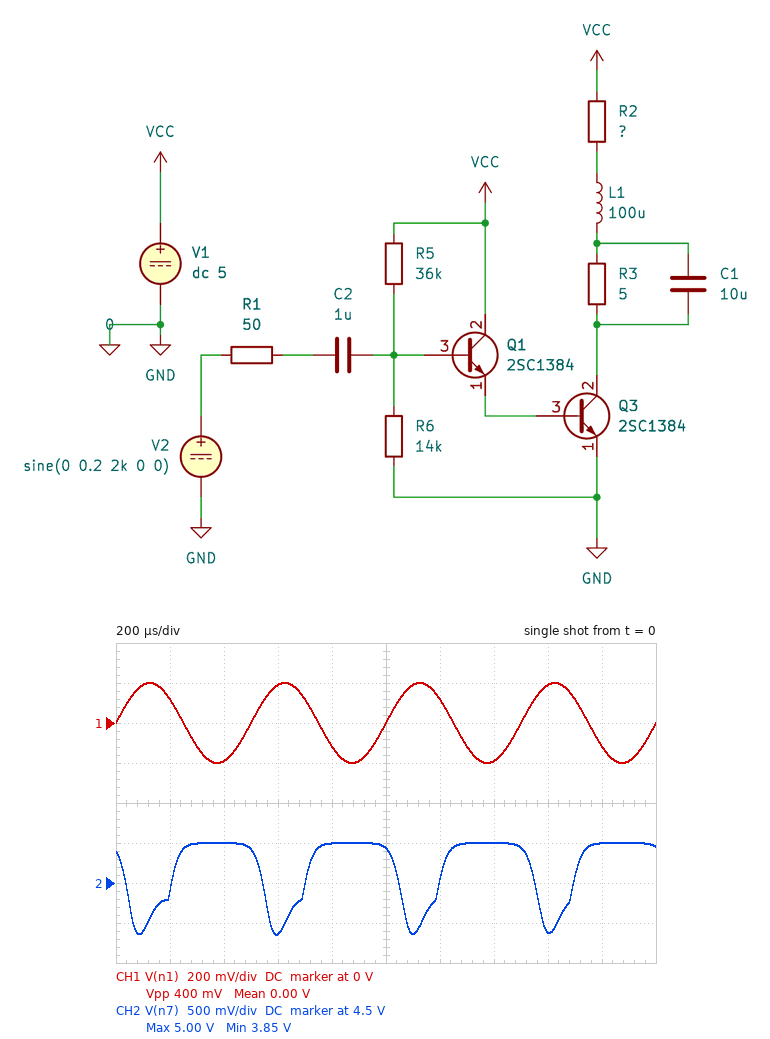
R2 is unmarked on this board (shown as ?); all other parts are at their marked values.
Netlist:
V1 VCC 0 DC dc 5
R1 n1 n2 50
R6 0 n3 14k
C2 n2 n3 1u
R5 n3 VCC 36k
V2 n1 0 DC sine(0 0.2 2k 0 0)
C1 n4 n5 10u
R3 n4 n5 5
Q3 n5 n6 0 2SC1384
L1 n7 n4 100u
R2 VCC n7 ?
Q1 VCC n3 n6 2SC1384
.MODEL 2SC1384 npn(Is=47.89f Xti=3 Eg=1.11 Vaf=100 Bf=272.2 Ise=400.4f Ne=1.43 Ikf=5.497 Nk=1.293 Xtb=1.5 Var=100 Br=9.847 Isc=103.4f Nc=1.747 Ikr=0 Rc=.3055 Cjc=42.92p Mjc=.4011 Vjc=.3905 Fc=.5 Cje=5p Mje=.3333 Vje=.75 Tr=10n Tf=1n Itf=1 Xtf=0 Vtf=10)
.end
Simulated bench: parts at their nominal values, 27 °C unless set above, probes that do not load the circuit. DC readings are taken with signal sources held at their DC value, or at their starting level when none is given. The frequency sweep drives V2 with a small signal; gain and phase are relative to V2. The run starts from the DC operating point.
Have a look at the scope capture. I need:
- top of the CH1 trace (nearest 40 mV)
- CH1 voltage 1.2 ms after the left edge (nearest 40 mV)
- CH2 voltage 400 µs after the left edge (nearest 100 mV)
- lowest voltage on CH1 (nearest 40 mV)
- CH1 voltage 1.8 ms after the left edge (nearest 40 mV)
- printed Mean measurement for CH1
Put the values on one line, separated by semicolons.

200 mV; 120 mV; 5.0 V; -200 mV; -120 mV; 0.00 V
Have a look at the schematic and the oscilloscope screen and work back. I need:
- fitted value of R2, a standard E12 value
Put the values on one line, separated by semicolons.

1 Ω
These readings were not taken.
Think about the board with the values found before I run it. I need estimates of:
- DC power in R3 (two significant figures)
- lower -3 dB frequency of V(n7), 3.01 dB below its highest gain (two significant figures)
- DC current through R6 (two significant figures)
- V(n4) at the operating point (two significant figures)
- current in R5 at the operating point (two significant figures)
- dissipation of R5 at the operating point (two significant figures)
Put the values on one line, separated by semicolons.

59 mW; 250 kHz; 95 µA; 4.9 V; 100 µA; 370 µW
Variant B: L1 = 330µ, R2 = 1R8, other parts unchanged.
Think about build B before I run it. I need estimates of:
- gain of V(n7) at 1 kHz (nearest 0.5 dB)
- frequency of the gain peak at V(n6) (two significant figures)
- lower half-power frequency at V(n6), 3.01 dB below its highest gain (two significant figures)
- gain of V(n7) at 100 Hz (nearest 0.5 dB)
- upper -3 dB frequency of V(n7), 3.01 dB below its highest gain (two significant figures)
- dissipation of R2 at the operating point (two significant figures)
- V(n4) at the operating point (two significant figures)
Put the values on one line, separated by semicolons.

11.5 dB; 200 kHz; 120 kHz; 11.0 dB; 260 kHz; 21 mW; 4.8 V
